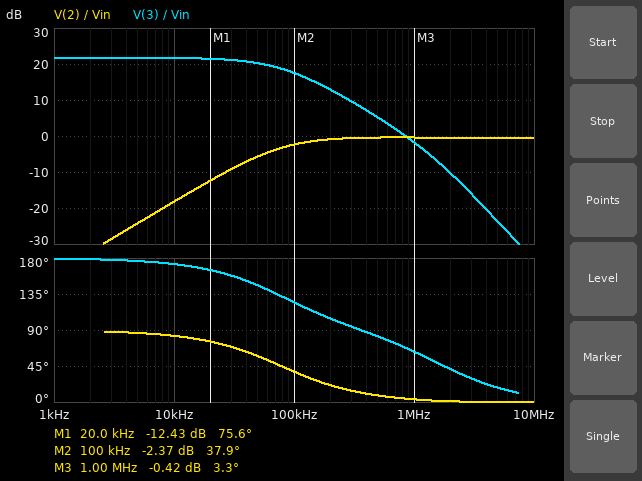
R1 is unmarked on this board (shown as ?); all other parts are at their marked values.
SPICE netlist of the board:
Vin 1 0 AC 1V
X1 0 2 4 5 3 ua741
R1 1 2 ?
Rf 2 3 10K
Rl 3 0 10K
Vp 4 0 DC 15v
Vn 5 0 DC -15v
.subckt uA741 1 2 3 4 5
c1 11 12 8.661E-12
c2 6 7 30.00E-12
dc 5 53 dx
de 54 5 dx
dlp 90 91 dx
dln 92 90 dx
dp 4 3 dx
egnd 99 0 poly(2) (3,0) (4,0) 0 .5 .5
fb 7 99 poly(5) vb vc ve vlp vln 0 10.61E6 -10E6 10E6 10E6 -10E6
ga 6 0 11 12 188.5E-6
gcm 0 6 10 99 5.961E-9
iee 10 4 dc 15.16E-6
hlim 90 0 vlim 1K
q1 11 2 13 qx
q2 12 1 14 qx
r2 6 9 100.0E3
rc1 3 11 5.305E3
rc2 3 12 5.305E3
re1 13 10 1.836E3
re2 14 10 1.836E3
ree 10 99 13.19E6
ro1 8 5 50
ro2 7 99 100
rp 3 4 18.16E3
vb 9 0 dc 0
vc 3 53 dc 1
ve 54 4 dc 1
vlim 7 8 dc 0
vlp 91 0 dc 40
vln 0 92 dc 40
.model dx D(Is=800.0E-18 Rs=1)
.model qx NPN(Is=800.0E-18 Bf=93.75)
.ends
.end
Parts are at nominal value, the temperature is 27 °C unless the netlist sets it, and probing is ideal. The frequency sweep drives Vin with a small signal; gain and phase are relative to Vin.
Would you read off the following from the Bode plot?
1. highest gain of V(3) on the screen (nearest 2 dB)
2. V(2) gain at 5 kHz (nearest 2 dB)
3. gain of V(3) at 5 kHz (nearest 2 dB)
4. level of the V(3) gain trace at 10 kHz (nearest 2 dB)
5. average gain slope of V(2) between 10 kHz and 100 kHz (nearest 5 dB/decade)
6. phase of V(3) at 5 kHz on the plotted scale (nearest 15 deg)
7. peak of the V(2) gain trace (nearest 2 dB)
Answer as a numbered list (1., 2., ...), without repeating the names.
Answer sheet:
1. 22 dB
2. -24 dB
3. 22 dB
4. 22 dB
5. 15 dB/decade
6. 180 deg
7. 0 dB
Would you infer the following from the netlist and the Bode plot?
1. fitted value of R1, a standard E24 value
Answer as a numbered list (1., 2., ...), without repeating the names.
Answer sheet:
1. 820 Ω
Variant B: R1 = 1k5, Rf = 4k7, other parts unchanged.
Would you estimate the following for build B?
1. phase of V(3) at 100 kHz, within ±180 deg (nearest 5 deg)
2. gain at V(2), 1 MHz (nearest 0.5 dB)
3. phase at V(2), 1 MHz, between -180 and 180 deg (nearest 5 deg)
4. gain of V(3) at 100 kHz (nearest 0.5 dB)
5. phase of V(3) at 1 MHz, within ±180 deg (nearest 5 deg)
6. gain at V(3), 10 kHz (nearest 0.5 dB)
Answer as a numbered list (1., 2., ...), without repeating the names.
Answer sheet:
1. 155 deg
2. -1.5 dB
3. 10 deg
4. 9.5 dB
5. 70 deg
6. 10.0 dB
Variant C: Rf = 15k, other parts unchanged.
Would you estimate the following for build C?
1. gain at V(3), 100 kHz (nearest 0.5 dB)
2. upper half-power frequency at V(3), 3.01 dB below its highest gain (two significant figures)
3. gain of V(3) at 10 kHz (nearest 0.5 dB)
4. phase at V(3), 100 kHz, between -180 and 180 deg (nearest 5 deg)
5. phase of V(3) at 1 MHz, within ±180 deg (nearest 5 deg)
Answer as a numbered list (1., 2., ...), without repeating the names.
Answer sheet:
1. 18.5 dB
2. 53 kHz
3. 25.0 dB
4. 115 deg
5. 60 deg
